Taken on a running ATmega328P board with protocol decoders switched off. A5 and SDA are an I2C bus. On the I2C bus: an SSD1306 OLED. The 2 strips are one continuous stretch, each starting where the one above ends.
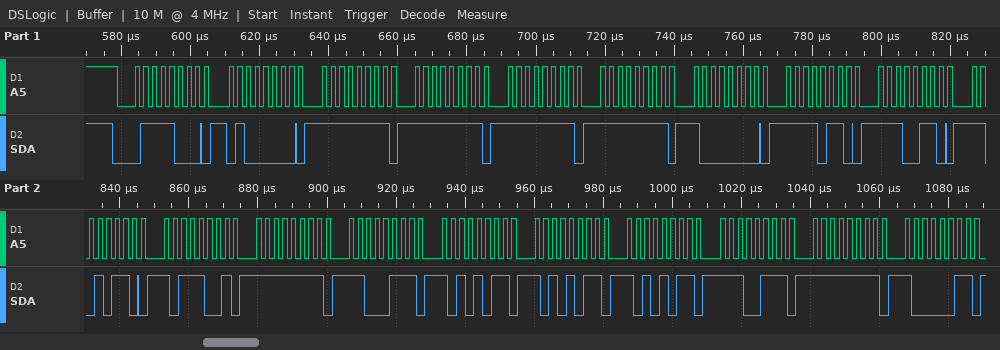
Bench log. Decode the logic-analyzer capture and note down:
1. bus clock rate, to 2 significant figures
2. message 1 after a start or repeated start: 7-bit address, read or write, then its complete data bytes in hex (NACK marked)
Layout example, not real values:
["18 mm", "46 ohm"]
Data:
["400 kHz", "0x3C write: 40 FF FF FF FF 80 F6 E6 D6 B9 FF C7 AB AB AB E7 FF 83"]
